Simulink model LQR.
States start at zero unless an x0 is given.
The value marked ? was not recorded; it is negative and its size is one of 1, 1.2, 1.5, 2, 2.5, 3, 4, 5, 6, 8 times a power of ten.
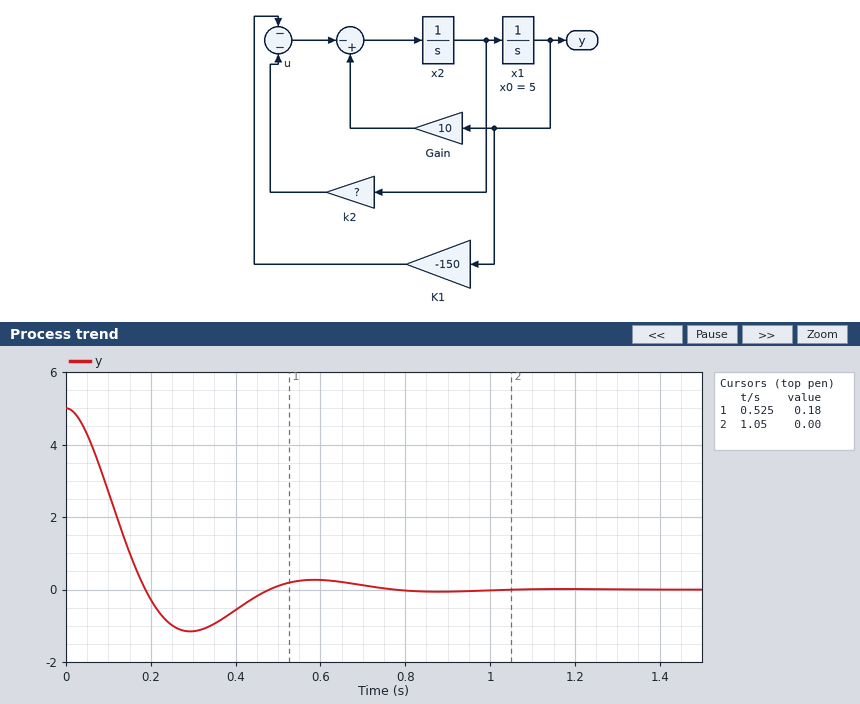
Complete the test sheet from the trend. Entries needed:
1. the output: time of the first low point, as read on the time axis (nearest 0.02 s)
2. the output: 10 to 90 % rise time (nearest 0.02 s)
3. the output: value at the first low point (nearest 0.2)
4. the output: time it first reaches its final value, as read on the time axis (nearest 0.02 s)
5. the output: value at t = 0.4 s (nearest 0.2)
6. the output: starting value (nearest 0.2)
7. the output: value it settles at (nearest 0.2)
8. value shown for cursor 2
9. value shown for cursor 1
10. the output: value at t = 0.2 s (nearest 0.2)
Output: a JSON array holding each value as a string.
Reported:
["0.30 s", "0.12 s", "-1.2", "0.18 s", "-0.6", "5.0", "0.0", "0.00", "0.18", "-0.2"]
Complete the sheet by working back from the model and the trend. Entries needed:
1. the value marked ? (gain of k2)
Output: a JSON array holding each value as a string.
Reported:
["-10"]
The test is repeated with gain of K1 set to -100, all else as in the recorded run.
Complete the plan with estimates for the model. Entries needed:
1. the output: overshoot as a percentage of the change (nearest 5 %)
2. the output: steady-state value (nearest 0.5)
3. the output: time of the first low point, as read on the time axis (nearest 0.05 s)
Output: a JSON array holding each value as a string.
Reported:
["15 %", "0.0", "0.40 s"]
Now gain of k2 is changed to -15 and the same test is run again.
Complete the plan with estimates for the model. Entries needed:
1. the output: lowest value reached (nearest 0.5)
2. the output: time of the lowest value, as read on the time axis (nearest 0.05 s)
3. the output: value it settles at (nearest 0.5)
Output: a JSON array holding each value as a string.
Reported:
["-0.5", "0.35 s", "0.0"]
